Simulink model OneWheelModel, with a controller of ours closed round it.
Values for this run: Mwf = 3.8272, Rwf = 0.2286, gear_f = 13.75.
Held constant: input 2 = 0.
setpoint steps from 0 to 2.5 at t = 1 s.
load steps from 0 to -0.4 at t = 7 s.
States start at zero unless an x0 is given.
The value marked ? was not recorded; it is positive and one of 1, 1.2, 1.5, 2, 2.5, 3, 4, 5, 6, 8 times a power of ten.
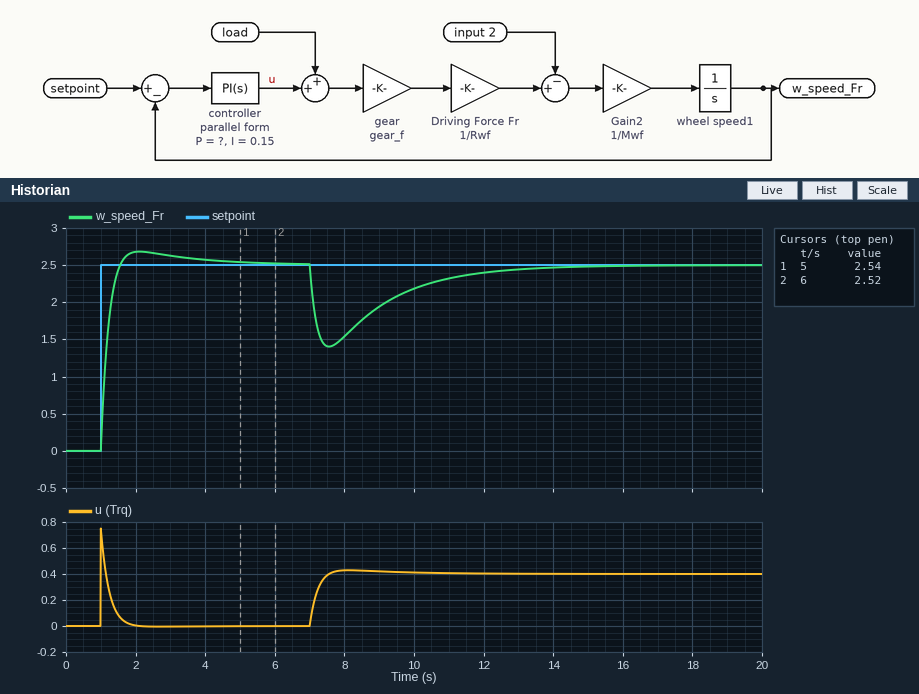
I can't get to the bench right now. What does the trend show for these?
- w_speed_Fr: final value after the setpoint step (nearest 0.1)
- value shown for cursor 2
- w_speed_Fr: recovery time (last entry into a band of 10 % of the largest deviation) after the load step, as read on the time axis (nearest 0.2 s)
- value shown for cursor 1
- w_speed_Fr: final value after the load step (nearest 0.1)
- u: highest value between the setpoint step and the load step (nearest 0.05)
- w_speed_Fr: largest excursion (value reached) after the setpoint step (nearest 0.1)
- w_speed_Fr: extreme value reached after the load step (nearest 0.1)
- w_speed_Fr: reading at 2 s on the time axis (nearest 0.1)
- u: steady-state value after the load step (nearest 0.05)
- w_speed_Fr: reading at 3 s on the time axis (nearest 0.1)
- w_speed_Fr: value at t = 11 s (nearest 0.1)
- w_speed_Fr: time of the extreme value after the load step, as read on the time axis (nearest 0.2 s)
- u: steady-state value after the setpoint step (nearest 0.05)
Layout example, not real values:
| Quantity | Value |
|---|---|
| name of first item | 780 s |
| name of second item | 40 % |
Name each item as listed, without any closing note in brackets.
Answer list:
| Quantity | Value |
|---|---|
| w_speed_Fr: final value after the setpoint step | 2.5 |
| value shown for cursor 2 | 2.52 |
| w_speed_Fr: recovery time (last entry into a band of 10 % of the largest deviation) after the load step, as read on the time axis | 11.8 s |
| value shown for cursor 1 | 2.54 |
| w_speed_Fr: final value after the load step | 2.5 |
| u: highest value between the setpoint step and the load step | 0.75 |
| w_speed_Fr: largest excursion (value reached) after the setpoint step | 2.7 |
| w_speed_Fr: extreme value reached after the load step | 1.4 |
| w_speed_Fr: reading at 2 s on the time axis | 2.7 |
| u: steady-state value after the load step | 0.40 |
| w_speed_Fr: reading at 3 s on the time axis | 2.6 |
| w_speed_Fr: value at t = 11 s | 2.3 |
| w_speed_Fr: time of the extreme value after the load step, as read on the time axis | 7.6 s |
| u: steady-state value after the setpoint step | 0.00 |
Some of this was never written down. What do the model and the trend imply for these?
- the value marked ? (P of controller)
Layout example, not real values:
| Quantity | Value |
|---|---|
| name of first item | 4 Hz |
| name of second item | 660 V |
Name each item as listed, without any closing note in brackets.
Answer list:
| Quantity | Value |
|---|---|
| the value marked ? | 0.3 |
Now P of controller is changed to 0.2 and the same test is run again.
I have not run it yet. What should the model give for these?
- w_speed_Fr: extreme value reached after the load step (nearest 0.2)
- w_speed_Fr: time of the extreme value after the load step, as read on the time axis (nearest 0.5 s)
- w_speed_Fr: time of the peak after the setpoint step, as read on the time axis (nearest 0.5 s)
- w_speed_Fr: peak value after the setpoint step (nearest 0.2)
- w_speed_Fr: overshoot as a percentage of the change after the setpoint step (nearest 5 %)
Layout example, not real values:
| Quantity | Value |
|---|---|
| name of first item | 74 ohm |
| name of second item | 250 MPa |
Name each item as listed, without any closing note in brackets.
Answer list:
| Quantity | Value |
|---|---|
| w_speed_Fr: extreme value reached after the load step | 1.0 |
| w_speed_Fr: time of the extreme value after the load step, as read on the time axis | 7.5 s |
| w_speed_Fr: time of the peak after the setpoint step, as read on the time axis | 2.5 s |
| w_speed_Fr: peak value after the setpoint step | 2.8 |
| w_speed_Fr: overshoot as a percentage of the change after the setpoint step | 15 % |
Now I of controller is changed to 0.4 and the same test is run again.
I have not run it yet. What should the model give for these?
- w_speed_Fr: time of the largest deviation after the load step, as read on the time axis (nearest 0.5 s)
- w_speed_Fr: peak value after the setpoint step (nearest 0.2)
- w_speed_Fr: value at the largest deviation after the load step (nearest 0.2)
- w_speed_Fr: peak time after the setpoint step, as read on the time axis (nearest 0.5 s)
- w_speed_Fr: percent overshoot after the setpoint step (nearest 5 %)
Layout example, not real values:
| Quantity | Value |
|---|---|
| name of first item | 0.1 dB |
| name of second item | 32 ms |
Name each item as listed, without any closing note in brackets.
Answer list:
| Quantity | Value |
|---|---|
| w_speed_Fr: time of the largest deviation after the load step, as read on the time axis | 7.5 s |
| w_speed_Fr: peak value after the setpoint step | 2.8 |
| w_speed_Fr: value at the largest deviation after the load step | 1.6 |
| w_speed_Fr: peak time after the setpoint step, as read on the time axis | 2.0 s |
| w_speed_Fr: percent overshoot after the setpoint step | 15 % |
